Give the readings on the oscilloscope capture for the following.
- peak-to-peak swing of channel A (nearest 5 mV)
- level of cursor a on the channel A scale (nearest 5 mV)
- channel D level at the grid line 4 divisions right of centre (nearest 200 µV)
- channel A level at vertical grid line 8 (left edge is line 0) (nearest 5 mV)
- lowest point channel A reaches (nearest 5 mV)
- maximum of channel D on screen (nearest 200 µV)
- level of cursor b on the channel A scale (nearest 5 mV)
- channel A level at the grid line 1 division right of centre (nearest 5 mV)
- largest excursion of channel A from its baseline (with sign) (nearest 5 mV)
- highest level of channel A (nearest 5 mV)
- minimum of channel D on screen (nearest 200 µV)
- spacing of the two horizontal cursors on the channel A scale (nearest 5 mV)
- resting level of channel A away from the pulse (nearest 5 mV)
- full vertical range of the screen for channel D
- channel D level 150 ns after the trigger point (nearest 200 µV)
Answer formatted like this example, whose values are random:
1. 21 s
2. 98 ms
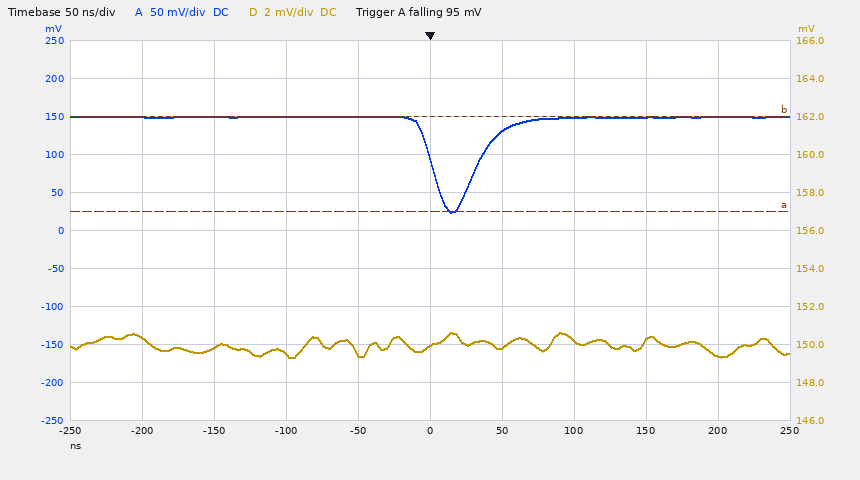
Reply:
1. 125 mV
2. 25 mV
3. 149.4 mV
4. 150 mV
5. 25 mV
6. 150.6 mV
7. 150 mV
8. 130 mV
9. -125 mV
10. 150 mV
11. 149.4 mV
12. 125 mV
13. 150 mV
14. 20 mV
15. 150.2 mV
